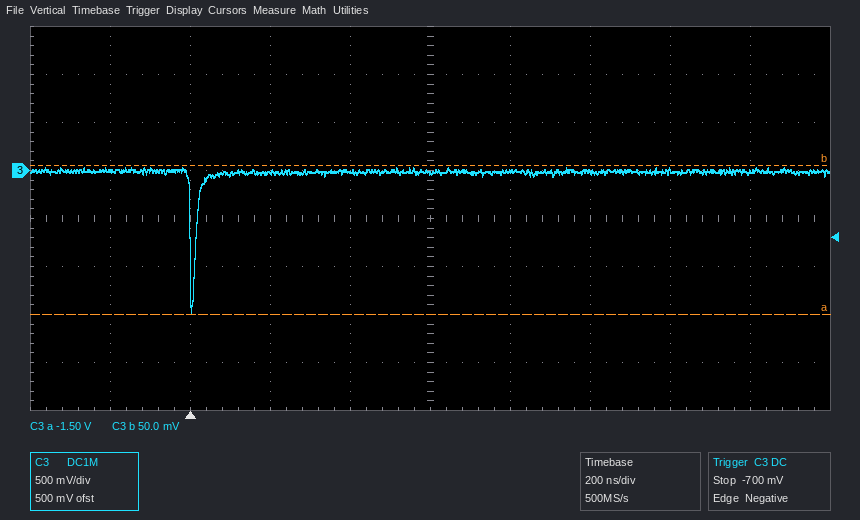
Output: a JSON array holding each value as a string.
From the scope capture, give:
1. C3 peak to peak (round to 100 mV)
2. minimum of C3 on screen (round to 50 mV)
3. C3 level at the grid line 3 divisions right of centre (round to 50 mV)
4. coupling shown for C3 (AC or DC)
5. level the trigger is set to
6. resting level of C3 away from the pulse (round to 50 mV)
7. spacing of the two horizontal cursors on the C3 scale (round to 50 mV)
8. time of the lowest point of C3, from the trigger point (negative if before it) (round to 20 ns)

["1.50 V", "-1.50 V", "0 mV", "DC", "-700 mV", "0 mV", "1.55 V", "0 ns"]
